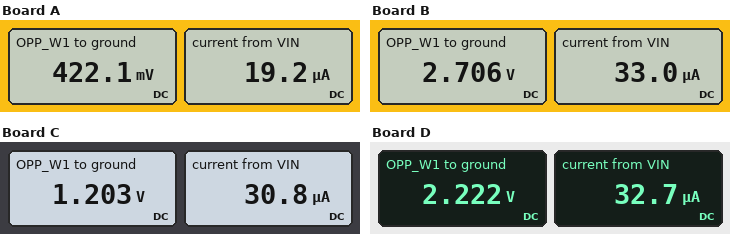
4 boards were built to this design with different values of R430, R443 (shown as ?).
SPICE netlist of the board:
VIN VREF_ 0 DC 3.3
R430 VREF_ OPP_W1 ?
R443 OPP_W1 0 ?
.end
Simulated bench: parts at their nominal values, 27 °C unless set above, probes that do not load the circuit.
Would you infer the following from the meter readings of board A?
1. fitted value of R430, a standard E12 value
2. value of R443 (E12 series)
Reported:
150 kΩ
22 kΩ
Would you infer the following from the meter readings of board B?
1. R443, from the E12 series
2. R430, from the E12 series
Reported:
82 kΩ
18 kΩ
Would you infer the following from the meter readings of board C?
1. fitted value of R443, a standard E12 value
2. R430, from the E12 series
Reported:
39 kΩ
68 kΩ
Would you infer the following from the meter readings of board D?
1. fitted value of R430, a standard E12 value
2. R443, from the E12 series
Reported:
33 kΩ
68 kΩ
